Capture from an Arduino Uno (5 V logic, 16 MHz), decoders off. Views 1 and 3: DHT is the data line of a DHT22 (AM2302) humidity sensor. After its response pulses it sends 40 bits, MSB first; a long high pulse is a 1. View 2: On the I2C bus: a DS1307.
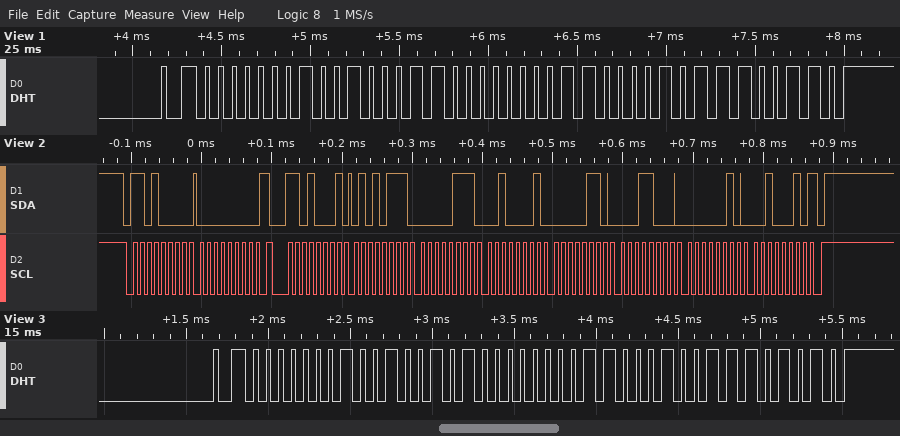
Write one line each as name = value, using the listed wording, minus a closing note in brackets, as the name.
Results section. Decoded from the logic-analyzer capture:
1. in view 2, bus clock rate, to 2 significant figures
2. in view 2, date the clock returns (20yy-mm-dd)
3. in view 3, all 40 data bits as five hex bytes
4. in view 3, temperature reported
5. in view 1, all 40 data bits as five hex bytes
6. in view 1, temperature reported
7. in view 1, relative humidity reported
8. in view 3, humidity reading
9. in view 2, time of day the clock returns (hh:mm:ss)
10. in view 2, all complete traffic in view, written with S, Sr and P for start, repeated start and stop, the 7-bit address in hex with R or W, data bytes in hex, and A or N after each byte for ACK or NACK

in view 2, bus clock rate, to 2 significant figures = 100 kHz
in view 2, date the clock returns = 2022-02-18
in view 3, all 40 data bits as five hex bytes = 01 25 00 C4 EA
in view 3, temperature reported = 19.6 °C
in view 1, all 40 data bits as five hex bytes = 01 23 00 C2 E6
in view 1, temperature reported = 19.4 °C
in view 1, relative humidity reported = 29.1 %
in view 3, humidity reading = 29.3 %
in view 2, time of day the clock returns = 21:07:57
in view 2, all complete traffic in view, written with S, Sr and P for start, repeated start and stop, the 7-bit address in hex with R or W, data bytes in hex, and A or N after each byte for ACK or NACK = S 68W A 00 A Sr 68R A 57 A 07 A 21 A 06 A 18 A 02 A 22 N P
